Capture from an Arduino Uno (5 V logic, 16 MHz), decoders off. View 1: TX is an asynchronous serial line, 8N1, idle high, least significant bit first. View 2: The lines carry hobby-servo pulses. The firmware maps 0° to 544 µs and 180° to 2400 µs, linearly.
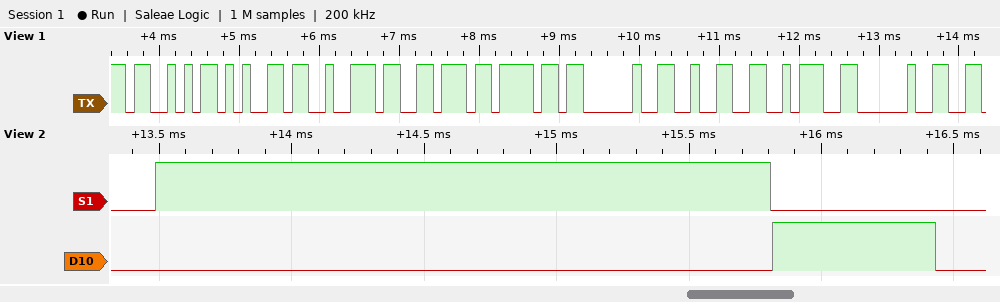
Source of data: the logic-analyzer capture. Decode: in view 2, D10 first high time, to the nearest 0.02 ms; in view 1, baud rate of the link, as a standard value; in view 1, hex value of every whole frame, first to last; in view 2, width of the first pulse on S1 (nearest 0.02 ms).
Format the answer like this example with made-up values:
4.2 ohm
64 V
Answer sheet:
0.62 ms
9600 baud
53 65 72 76 6F 20 32 3A 20
2.32 ms
